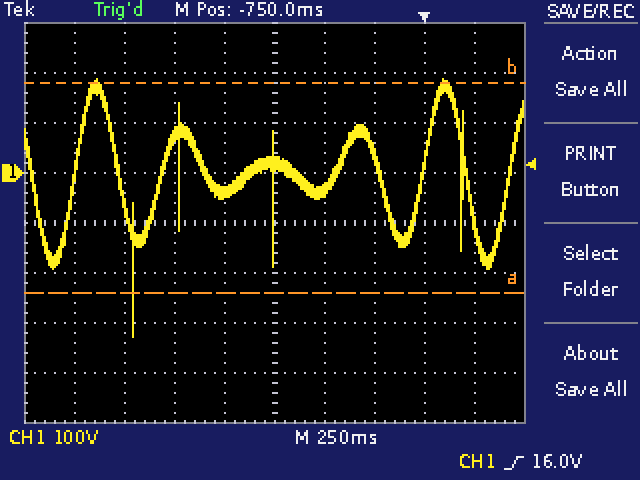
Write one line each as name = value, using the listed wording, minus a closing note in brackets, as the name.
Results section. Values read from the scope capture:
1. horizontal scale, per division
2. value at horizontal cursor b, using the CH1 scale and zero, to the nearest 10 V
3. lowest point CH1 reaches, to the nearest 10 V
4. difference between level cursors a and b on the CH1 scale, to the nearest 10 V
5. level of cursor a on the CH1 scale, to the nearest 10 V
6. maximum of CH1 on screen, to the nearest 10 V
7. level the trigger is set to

horizontal scale, per division = 250 ms
value at horizontal cursor b, using the CH1 scale and zero, to the nearest 10 V = 180 V
lowest point CH1 reaches, to the nearest 10 V = -330 V
difference between level cursors a and b on the CH1 scale, to the nearest 10 V = 420 V
level of cursor a on the CH1 scale, to the nearest 10 V = -240 V
maximum of CH1 on screen, to the nearest 10 V = 190 V
level the trigger is set to = 16.0 V
